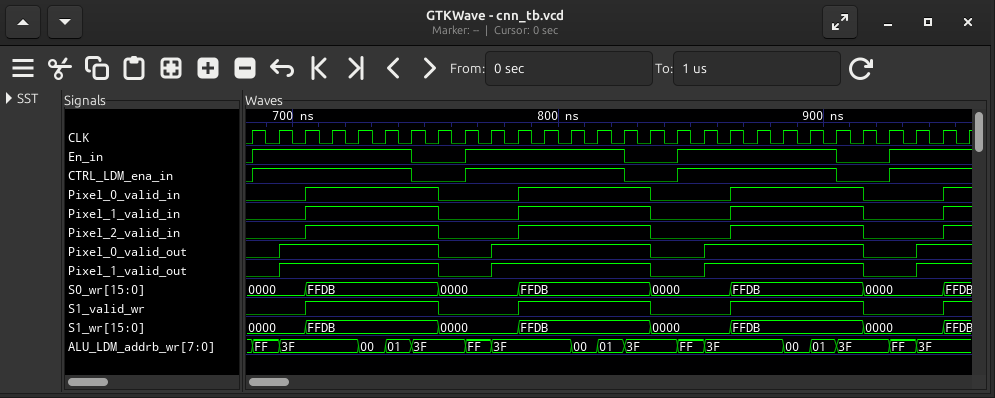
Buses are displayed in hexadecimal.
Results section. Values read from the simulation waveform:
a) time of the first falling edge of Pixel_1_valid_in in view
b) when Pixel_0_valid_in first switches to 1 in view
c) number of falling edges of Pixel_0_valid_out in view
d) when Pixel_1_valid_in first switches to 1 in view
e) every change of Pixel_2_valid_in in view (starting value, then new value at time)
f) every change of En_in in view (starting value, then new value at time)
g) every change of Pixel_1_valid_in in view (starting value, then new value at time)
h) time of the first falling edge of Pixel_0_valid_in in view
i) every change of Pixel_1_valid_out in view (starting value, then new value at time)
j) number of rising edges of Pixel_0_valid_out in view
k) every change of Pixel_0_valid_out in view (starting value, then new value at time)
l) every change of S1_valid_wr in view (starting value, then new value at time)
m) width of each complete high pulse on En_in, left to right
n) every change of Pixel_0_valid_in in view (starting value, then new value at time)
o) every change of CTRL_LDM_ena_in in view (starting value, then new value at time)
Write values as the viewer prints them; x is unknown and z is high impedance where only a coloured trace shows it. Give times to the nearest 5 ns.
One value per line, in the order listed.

755 ns
705 ns
3
705 ns
0, 1 at 705 ns, 0 at 755 ns, 1 at 785 ns, 0 at 835 ns, 1 at 865 ns, 0 at 915 ns, 1 at 945 ns
0, 1 at 685 ns, 0 at 745 ns, 1 at 765 ns, 0 at 825 ns, 1 at 845 ns, 0 at 905 ns, 1 at 925 ns
0, 1 at 705 ns, 0 at 755 ns, 1 at 785 ns, 0 at 835 ns, 1 at 865 ns, 0 at 915 ns, 1 at 945 ns
755 ns
0, 1 at 695 ns, 0 at 755 ns, 1 at 775 ns, 0 at 835 ns, 1 at 855 ns, 0 at 915 ns, 1 at 935 ns
4
0, 1 at 695 ns, 0 at 755 ns, 1 at 775 ns, 0 at 835 ns, 1 at 855 ns, 0 at 915 ns, 1 at 935 ns
0, 1 at 705 ns, 0 at 755 ns, 1 at 785 ns, 0 at 835 ns, 1 at 865 ns, 0 at 915 ns, 1 at 945 ns
60 ns, 60 ns, 60 ns
0, 1 at 705 ns, 0 at 755 ns, 1 at 785 ns, 0 at 835 ns, 1 at 865 ns, 0 at 915 ns, 1 at 945 ns
0, 1 at 685 ns, 0 at 745 ns, 1 at 765 ns, 0 at 825 ns, 1 at 845 ns, 0 at 905 ns, 1 at 925 ns
